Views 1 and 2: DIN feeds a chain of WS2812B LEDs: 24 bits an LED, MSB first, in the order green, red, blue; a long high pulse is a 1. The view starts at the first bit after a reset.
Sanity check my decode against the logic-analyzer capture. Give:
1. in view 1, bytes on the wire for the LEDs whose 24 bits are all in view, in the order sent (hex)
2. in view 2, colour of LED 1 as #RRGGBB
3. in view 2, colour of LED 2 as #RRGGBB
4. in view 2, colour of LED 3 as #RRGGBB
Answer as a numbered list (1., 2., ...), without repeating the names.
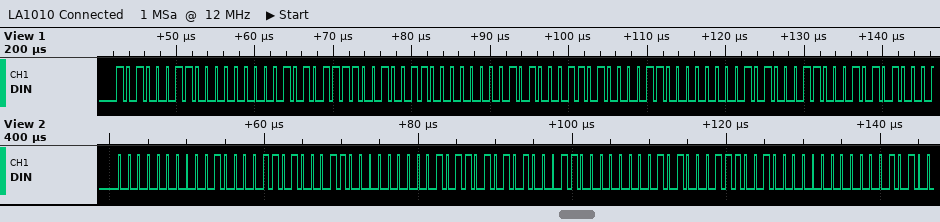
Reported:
1. A3 00 57 93 00 A3 43 00 A3
2. #2100A3
3. #5A00A3
4. #A30090
